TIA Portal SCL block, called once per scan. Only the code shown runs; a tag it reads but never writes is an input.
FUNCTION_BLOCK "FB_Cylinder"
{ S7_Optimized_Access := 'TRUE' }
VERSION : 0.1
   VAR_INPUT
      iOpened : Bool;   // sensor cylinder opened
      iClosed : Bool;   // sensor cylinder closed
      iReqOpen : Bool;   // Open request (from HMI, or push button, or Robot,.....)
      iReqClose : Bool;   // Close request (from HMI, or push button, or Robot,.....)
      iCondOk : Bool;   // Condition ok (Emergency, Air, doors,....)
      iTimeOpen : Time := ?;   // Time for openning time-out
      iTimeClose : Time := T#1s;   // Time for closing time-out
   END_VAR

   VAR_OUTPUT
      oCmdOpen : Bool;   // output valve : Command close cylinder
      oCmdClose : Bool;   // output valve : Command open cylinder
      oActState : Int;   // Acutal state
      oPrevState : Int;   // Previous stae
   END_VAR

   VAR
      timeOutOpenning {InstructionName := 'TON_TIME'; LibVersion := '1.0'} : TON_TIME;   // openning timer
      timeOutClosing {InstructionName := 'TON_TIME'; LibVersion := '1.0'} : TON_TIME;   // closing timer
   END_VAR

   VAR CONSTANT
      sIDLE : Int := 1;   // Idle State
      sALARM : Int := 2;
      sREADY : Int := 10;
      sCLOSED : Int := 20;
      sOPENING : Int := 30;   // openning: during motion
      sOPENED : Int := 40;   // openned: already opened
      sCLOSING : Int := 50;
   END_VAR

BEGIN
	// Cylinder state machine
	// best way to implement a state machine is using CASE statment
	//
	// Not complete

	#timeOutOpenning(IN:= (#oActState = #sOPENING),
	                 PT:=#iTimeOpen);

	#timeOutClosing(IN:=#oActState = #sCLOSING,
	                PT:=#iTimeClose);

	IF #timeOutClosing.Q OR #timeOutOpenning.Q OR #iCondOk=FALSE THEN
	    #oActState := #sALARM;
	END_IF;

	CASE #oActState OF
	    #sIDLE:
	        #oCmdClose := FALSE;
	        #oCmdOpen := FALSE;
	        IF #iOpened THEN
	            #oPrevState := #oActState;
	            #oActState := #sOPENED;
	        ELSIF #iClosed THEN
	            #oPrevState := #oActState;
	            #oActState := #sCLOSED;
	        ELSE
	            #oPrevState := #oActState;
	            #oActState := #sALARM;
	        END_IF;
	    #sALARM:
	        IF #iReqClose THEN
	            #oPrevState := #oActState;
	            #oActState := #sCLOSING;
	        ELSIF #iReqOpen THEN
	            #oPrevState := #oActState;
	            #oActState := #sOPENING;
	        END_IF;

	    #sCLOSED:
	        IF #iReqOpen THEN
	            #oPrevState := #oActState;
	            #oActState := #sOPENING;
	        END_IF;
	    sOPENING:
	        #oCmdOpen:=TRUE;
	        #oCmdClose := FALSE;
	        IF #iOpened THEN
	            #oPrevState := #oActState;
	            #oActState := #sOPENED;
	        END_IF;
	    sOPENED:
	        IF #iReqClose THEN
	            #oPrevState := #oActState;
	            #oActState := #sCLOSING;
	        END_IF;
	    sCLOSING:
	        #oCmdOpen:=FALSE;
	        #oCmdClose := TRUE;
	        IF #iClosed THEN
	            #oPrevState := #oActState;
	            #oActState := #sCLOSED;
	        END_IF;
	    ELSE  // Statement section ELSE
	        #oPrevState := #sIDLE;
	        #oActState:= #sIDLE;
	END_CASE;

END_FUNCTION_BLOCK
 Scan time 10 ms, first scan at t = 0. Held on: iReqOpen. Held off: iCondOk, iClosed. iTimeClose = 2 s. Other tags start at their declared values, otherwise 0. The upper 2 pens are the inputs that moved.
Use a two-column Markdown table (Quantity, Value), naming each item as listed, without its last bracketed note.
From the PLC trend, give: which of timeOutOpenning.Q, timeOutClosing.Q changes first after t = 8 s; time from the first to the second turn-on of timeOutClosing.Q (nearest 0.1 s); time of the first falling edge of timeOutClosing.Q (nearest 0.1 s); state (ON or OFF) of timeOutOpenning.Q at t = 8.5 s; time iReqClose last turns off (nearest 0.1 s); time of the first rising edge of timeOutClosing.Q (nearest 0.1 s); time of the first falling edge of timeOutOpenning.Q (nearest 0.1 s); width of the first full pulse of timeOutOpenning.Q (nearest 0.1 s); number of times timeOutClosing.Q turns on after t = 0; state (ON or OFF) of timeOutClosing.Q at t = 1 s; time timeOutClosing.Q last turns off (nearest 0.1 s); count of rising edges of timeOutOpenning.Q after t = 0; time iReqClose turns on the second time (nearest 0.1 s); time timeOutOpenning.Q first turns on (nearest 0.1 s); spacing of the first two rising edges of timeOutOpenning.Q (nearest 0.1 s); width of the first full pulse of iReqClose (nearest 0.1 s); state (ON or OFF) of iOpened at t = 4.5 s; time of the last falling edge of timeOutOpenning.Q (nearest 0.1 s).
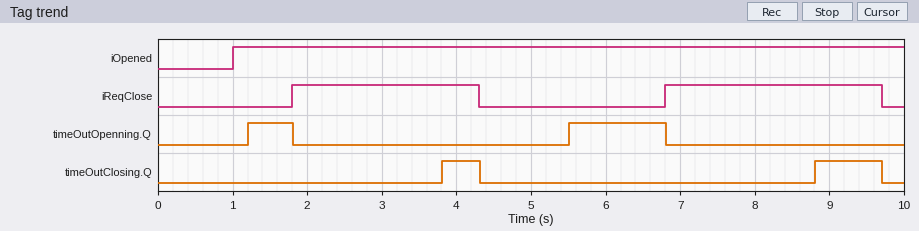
| Quantity | Value |
|---|---|
| which of timeOutOpenning.Q, timeOutClosing.Q changes first after t = 8 s | timeOutClosing.Q |
| time from the first to the second turn-on of timeOutClosing.Q | 5.0 s |
| time of the first falling edge of timeOutClosing.Q | 4.3 s |
| state (ON or OFF) of timeOutOpenning.Q at t = 8.5 s | OFF |
| time iReqClose last turns off | 9.7 s |
| time of the first rising edge of timeOutClosing.Q | 3.8 s |
| time of the first falling edge of timeOutOpenning.Q | 1.8 s |
| width of the first full pulse of timeOutOpenning.Q | 0.6 s |
| number of times timeOutClosing.Q turns on after t = 0 | 2 |
| state (ON or OFF) of timeOutClosing.Q at t = 1 s | OFF |
| time timeOutClosing.Q last turns off | 9.7 s |
| count of rising edges of timeOutOpenning.Q after t = 0 | 2 |
| time iReqClose turns on the second time | 6.8 s |
| time timeOutOpenning.Q first turns on | 1.2 s |
| spacing of the first two rising edges of timeOutOpenning.Q | 4.3 s |
| width of the first full pulse of iReqClose | 2.5 s |
| state (ON or OFF) of iOpened at t = 4.5 s | ON |
| time of the last falling edge of timeOutOpenning.Q | 6.8 s |
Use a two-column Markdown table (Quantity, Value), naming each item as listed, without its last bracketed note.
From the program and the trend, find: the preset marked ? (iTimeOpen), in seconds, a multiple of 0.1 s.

| Quantity | Value |
|---|---|
| the preset marked ? (iTimeOpen), in seconds, a multiple of 0.1 s | 1.2 s |
